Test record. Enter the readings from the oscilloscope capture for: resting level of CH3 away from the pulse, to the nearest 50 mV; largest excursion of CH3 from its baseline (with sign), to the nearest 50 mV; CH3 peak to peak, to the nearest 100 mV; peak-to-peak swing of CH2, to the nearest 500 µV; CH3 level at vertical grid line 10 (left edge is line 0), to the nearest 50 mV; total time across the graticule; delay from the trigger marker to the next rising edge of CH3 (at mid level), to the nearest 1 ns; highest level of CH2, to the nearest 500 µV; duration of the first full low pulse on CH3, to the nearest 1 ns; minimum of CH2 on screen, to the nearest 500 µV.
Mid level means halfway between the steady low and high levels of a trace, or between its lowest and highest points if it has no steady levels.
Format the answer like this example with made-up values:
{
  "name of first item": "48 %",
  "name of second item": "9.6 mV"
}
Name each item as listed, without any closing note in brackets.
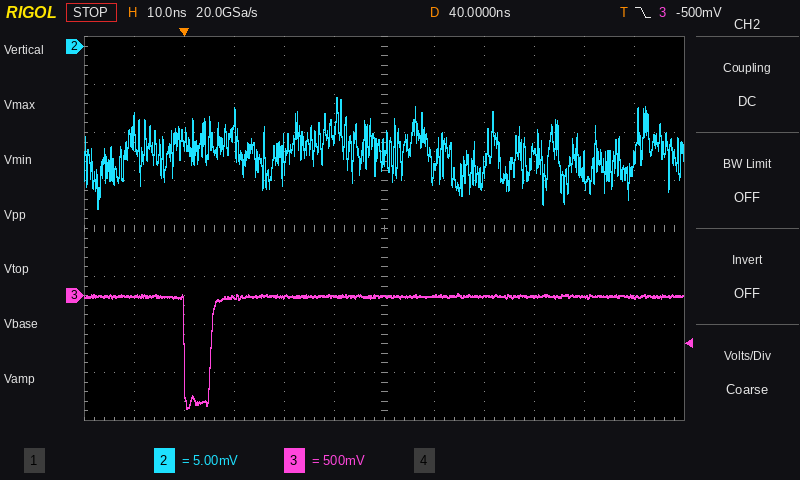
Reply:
{
  "resting level of CH3 away from the pulse, to the nearest 50 mV": "0 mV",
  "largest excursion of CH3 from its baseline (with sign), to the nearest 50 mV": "-1.15 V",
  "CH3 peak to peak, to the nearest 100 mV": "1.20 V",
  "peak-to-peak swing of CH2, to the nearest 500 µV": "11.5 mV",
  "CH3 level at vertical grid line 10 (left edge is line 0), to the nearest 50 mV": "0 mV",
  "total time across the graticule": "120 ns",
  "delay from the trigger marker to the next rising edge of CH3 (at mid level), to the nearest 1 ns": "5 ns",
  "highest level of CH2, to the nearest 500 µV": "-5.5 mV",
  "duration of the first full low pulse on CH3, to the nearest 1 ns": "5 ns",
  "minimum of CH2 on screen, to the nearest 500 µV": "-17.0 mV"
}
